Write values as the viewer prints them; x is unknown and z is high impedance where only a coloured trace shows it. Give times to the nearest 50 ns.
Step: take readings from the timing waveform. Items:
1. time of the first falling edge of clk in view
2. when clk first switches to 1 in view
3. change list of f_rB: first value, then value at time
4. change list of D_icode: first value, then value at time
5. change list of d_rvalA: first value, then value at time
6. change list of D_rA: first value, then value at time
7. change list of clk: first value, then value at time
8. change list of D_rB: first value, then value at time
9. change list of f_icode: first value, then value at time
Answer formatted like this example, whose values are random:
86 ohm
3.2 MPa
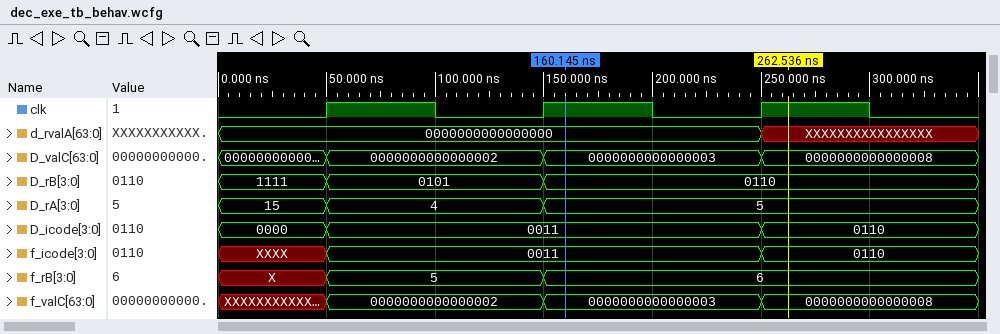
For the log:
100 ns
50 ns
X, 5 at 50 ns, 6 at 150 ns
0000, 0011 at 50 ns, 0110 at 250 ns
0000000000000000, XXXXXXXXXXXXXXXX at 250 ns
15, 4 at 50 ns, 5 at 150 ns
0, 1 at 50 ns, 0 at 100 ns, 1 at 150 ns, 0 at 200 ns, 1 at 250 ns, 0 at 300 ns
1111, 0101 at 50 ns, 0110 at 150 ns
XXXX, 0011 at 50 ns, 0110 at 250 ns
